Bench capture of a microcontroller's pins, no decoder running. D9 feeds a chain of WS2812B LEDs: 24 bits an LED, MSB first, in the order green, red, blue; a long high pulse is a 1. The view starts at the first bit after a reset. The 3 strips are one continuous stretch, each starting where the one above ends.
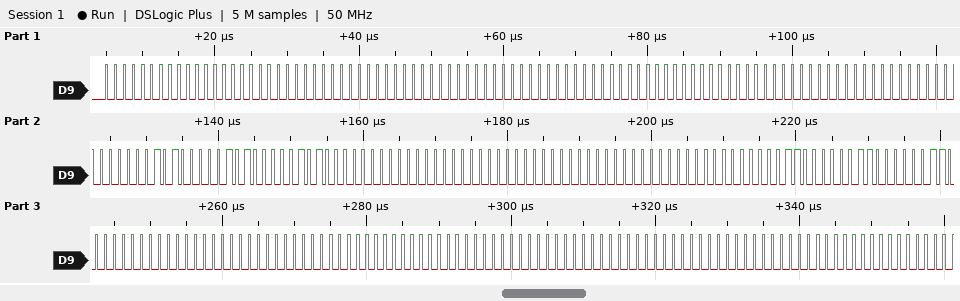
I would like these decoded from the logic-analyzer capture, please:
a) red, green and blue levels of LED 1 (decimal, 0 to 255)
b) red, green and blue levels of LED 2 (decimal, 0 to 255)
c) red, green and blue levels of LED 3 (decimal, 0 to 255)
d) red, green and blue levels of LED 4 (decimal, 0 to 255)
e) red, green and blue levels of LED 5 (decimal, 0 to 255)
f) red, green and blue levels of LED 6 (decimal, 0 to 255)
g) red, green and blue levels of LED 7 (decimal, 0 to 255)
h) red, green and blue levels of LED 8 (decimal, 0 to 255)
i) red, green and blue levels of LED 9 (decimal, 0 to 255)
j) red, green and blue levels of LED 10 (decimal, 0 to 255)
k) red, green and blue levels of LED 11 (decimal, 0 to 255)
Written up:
0, 0, 0
0, 0, 0
0, 0, 0
0, 0, 0
5, 5, 5
0, 0, 0
0, 0, 0
24, 24, 24
0, 0, 0
0, 0, 0
0, 0, 0
